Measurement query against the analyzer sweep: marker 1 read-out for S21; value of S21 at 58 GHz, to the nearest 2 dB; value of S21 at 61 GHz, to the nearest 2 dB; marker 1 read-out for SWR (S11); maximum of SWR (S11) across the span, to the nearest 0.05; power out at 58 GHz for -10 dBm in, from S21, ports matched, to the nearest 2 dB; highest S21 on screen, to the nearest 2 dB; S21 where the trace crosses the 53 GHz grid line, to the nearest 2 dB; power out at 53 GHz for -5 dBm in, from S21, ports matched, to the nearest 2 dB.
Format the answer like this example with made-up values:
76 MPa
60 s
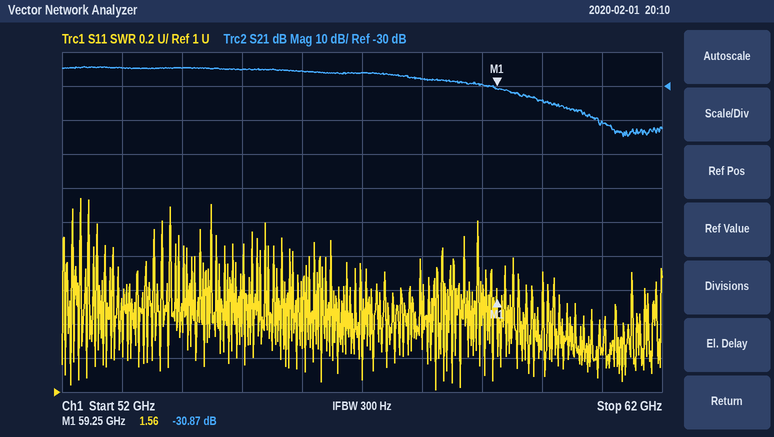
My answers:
-30.87 dB
-28 dB
-40 dB
1.56
2.15
-38 dBm
-24 dB
-24 dB
-30 dBm
